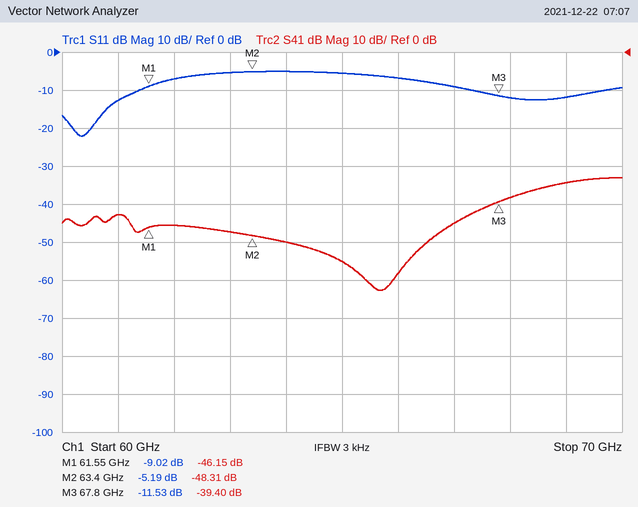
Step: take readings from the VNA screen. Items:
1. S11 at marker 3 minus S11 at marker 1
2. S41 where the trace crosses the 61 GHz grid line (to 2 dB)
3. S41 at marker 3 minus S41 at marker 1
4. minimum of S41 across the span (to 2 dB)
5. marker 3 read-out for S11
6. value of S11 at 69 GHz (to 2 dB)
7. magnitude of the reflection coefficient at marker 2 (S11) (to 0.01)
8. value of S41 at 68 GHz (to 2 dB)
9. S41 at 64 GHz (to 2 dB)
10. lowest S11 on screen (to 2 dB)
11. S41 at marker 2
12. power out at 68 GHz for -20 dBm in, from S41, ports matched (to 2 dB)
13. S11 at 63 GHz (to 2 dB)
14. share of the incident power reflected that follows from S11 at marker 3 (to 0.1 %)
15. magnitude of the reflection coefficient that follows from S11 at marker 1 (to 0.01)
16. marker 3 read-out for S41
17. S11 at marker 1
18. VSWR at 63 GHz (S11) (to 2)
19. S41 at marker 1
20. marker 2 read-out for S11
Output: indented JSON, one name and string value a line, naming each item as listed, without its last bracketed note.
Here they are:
{
  "S11 at marker 3 minus S11 at marker 1": "-2.51 dB",
  "S41 where the trace crosses the 61 GHz grid line": "-42 dB",
  "S41 at marker 3 minus S41 at marker 1": "6.75 dB",
  "minimum of S41 across the span": "-62 dB",
  "marker 3 read-out for S11": "-11.53 dB",
  "value of S11 at 69 GHz": "-12 dB",
  "magnitude of the reflection coefficient at marker 2 (S11)": "0.55",
  "value of S41 at 68 GHz": "-38 dB",
  "S41 at 64 GHz": "-50 dB",
  "lowest S11 on screen": "-22 dB",
  "S41 at marker 2": "-48.31 dB",
  "power out at 68 GHz for -20 dBm in, from S41, ports matched": "-58 dBm",
  "S11 at 63 GHz": "-6 dB",
  "share of the incident power reflected that follows from S11 at marker 3": "7.0 %",
  "magnitude of the reflection coefficient that follows from S11 at marker 1": "0.35",
  "marker 3 read-out for S41": "-39.40 dB",
  "S11 at marker 1": "-9.02 dB",
  "VSWR at 63 GHz (S11)": "4",
  "S41 at marker 1": "-46.15 dB",
  "marker 2 read-out for S11": "-5.19 dB"
}
